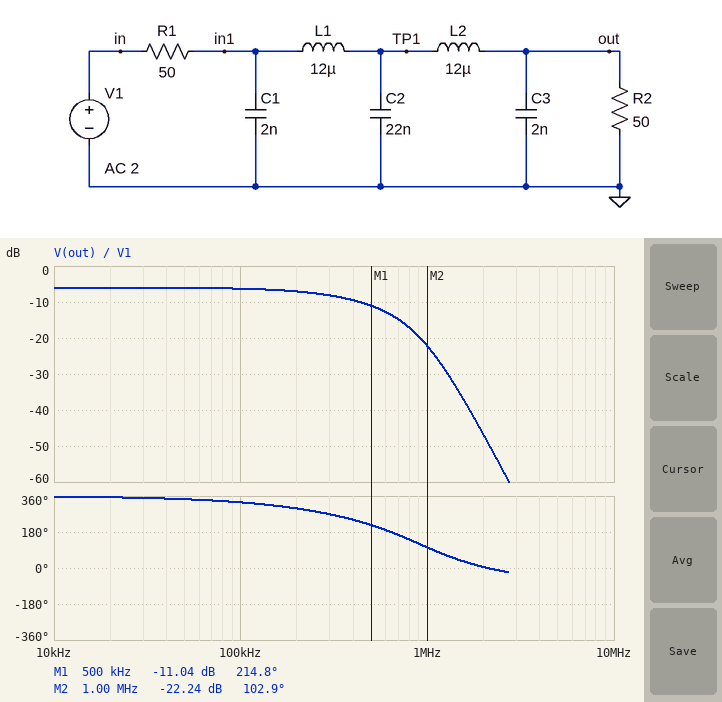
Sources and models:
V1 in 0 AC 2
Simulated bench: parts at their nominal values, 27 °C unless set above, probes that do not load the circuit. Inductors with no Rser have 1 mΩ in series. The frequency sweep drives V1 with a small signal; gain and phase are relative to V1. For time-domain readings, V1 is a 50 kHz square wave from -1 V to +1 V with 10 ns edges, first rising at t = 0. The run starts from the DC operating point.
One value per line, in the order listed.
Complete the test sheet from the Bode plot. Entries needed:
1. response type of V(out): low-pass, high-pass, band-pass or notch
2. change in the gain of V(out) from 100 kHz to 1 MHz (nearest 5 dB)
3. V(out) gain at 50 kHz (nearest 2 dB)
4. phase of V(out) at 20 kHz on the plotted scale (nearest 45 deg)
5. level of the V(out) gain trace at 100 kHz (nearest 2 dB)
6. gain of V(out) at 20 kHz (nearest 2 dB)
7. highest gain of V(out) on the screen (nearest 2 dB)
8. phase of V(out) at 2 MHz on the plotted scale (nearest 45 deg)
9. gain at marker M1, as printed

low-pass
-15 dB
-6 dB
360 deg
-6 dB
-6 dB
-6 dB
0 deg
-11.04 dB
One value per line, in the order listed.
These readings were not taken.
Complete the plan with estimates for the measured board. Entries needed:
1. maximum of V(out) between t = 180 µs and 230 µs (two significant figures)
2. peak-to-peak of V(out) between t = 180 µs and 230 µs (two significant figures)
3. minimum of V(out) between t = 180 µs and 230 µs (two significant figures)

500 mV
1.0 V
-500 mV
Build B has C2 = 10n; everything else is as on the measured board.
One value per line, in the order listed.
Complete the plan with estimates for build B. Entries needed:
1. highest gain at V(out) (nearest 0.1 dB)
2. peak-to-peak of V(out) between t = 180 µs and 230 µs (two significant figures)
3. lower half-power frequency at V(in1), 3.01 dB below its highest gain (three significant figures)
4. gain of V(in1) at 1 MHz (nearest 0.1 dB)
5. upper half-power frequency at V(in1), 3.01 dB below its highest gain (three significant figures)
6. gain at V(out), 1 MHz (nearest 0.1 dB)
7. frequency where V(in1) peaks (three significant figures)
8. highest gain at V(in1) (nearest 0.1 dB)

-6.0 dB
1.2 V
822 kHz
-0.7 dB
2.16 MHz
-13.4 dB
1.19 MHz
-0.1 dB
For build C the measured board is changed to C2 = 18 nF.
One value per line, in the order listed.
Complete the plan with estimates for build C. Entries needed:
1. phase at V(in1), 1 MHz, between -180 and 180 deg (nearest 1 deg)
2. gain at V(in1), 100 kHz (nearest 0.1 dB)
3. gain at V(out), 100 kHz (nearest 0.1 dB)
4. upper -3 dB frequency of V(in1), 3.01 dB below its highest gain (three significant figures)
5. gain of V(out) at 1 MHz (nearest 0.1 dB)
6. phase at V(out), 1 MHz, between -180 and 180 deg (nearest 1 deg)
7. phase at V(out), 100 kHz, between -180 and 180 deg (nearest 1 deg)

8 deg
-6.7 dB
-6.2 dB
2.12 MHz
-20.1 dB
105 deg
-28 deg
